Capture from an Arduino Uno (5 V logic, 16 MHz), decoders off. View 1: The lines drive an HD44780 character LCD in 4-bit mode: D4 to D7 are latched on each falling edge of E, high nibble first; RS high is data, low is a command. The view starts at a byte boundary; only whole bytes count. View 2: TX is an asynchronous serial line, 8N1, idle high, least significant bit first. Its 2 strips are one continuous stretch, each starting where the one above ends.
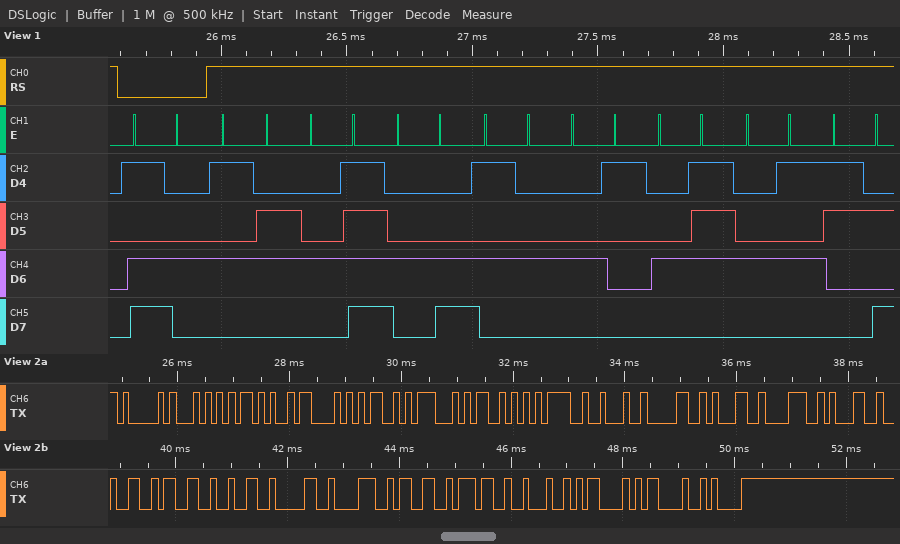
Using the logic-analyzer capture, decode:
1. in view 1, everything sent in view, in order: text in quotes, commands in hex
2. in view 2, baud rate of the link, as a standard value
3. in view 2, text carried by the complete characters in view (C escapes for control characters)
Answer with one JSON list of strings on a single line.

["0xD4 \"VOLTAGE:\"", "9600 baud", "\"AT+CMGS=\\\"01812320837\\\"\\r\\r\\n\""]
